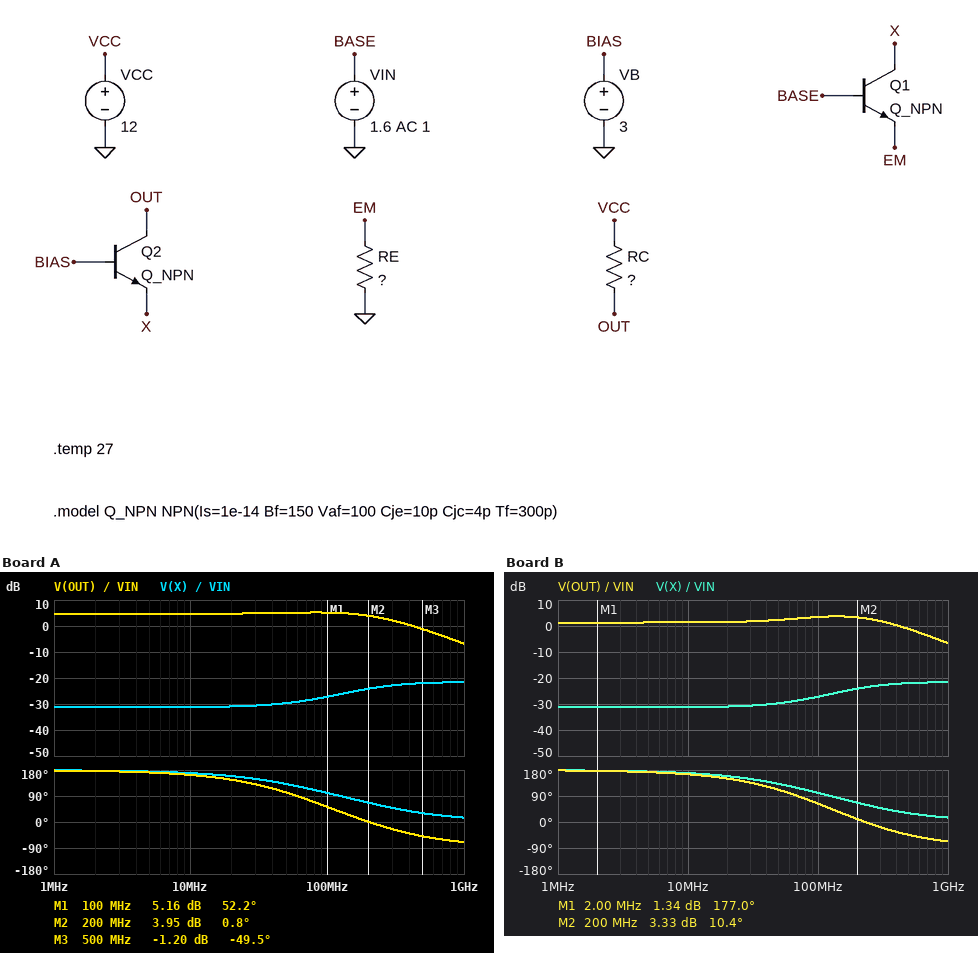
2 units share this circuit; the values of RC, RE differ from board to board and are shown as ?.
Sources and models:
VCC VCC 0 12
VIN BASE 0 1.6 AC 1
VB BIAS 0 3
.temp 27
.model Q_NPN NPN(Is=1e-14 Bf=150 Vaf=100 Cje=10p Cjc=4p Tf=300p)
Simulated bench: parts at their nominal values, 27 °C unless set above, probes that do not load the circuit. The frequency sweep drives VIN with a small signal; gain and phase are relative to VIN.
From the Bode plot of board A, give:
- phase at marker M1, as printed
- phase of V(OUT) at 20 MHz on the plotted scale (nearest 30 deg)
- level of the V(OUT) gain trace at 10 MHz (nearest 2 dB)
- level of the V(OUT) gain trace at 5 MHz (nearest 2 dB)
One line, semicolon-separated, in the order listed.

52.2 deg; 150 deg; 4 dB; 4 dB
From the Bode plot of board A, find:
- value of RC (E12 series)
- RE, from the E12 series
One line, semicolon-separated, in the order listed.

1 kΩ; 560 Ω
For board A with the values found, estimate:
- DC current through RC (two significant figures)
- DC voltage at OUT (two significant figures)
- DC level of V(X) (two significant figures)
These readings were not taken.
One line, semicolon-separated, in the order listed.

1.6 mA; 10 V; 2.3 V
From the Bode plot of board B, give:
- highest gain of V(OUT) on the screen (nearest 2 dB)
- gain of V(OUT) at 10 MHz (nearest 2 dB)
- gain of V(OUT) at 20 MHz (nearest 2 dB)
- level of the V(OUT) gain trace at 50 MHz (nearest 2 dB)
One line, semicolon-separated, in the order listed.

4 dB; 2 dB; 2 dB; 2 dB
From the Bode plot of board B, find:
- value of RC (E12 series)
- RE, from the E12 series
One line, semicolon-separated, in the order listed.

680 Ω; 560 Ω
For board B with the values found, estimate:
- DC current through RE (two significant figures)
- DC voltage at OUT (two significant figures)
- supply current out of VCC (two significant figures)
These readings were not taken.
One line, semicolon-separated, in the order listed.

1.7 mA; 11 V; 1.6 mA
